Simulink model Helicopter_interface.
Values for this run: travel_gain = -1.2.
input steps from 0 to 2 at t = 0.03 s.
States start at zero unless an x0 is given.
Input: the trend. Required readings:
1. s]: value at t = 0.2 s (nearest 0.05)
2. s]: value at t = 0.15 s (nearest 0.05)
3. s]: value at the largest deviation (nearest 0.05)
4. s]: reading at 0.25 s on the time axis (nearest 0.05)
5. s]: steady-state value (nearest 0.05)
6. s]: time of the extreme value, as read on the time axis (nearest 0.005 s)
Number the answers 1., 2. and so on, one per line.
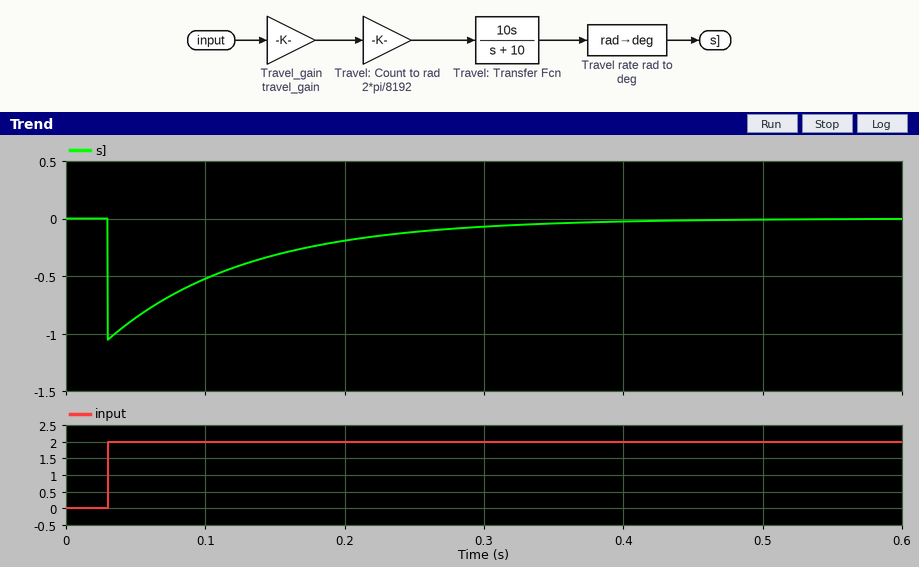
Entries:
1. -0.20
2. -0.30
3. -1.05
4. -0.10
5. 0.00
6. 0.030 s
